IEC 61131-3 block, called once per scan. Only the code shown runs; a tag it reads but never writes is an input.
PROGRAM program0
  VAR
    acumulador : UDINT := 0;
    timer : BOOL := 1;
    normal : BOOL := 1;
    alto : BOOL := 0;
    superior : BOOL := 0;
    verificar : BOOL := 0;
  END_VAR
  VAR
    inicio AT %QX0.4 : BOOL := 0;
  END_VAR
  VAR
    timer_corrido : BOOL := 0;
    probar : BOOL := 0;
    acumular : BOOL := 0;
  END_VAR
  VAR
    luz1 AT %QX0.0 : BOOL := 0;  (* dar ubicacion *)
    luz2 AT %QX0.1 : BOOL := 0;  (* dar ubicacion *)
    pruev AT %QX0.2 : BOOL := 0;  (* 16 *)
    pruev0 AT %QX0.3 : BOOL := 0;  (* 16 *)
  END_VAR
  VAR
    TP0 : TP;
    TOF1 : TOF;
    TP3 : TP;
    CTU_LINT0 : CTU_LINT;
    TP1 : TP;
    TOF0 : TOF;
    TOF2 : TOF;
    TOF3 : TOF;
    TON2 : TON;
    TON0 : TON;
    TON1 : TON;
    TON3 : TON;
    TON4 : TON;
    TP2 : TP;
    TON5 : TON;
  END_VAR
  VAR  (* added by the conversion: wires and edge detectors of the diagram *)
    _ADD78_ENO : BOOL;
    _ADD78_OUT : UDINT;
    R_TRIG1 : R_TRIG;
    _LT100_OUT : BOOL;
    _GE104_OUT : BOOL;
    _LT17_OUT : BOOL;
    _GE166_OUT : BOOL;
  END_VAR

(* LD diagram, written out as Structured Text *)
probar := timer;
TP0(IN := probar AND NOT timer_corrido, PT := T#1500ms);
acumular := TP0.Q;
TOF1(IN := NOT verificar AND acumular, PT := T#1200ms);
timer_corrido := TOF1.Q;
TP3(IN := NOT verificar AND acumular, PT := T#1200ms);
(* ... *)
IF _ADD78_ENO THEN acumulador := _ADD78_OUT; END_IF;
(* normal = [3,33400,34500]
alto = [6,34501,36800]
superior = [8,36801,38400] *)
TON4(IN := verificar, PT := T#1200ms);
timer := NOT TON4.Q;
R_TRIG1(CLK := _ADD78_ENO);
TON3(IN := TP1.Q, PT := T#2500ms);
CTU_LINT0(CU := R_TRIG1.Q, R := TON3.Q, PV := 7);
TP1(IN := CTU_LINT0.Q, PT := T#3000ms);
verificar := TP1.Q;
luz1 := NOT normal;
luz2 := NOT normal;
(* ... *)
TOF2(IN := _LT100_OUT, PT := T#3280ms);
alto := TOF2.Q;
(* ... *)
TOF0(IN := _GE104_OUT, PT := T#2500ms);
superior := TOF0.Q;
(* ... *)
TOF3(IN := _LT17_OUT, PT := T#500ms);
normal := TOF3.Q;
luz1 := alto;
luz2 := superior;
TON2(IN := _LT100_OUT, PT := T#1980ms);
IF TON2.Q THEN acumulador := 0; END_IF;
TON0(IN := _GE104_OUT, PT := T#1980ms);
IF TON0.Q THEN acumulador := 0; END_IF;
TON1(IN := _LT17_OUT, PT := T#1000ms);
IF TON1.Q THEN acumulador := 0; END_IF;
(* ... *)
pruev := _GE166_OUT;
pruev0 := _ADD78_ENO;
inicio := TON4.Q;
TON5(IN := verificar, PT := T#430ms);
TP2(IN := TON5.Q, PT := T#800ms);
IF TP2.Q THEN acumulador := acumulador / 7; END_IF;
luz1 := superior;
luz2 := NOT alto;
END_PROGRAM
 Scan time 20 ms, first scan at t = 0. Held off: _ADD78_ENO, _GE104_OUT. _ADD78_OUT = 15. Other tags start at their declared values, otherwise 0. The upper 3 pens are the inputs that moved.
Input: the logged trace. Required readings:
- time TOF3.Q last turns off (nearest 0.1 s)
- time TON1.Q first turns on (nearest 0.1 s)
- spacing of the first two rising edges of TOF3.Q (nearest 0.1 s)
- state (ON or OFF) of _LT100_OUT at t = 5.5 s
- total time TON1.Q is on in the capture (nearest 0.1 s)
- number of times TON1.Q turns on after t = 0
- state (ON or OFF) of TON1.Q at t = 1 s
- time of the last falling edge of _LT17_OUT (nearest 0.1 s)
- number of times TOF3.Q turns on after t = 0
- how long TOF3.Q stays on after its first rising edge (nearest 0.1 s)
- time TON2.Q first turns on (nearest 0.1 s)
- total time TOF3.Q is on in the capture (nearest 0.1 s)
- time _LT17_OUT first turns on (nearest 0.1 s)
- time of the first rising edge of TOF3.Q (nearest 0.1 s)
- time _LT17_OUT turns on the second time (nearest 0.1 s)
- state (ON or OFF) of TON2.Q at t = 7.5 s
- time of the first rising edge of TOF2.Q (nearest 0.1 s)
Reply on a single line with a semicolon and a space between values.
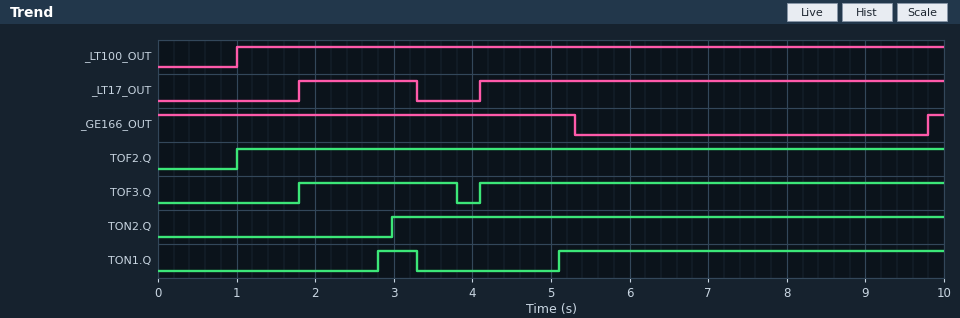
3.8 s; 2.8 s; 2.3 s; ON; 5.4 s; 2; OFF; 3.3 s; 2; 2.0 s; 3.0 s; 7.9 s; 1.8 s; 1.8 s; 4.1 s; ON; 1.0 s
